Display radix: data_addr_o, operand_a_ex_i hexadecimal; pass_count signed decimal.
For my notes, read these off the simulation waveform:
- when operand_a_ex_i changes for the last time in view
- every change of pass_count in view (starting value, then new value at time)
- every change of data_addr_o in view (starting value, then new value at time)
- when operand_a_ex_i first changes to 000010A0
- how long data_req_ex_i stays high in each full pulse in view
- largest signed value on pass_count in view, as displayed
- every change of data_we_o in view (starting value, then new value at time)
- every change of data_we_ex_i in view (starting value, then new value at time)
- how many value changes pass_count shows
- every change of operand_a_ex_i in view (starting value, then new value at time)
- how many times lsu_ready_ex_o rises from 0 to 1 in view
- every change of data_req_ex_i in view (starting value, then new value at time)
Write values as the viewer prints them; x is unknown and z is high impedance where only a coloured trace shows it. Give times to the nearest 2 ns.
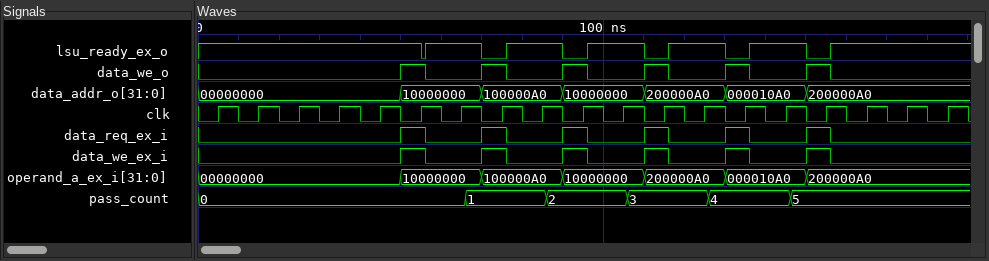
150 ns
0, 1 at 66 ns, 2 at 86 ns, 3 at 106 ns, 4 at 126 ns, 5 at 146 ns
00000000, 10000000 at 50 ns, 100000A0 at 70 ns, 10000000 at 90 ns, 200000A0 at 110 ns, 000010A0 at 130 ns, 200000A0 at 150 ns
130 ns
6 ns, 6 ns, 6 ns, 6 ns, 6 ns, 6 ns
5
0, 1 at 50 ns, 0 at 56 ns, 1 at 70 ns, 0 at 76 ns, 1 at 90 ns, 0 at 96 ns, 1 at 110 ns, 0 at 116 ns, 1 at 130 ns, 0 at 136 ns, 1 at 150 ns, 0 at 156 ns
0, 1 at 50 ns, 0 at 56 ns, 1 at 70 ns, 0 at 76 ns, 1 at 90 ns, 0 at 96 ns, 1 at 110 ns, 0 at 116 ns, 1 at 130 ns, 0 at 136 ns, 1 at 150 ns, 0 at 156 ns
5
00000000, 10000000 at 50 ns, 100000A0 at 70 ns, 10000000 at 90 ns, 200000A0 at 110 ns, 000010A0 at 130 ns, 200000A0 at 150 ns
6
0, 1 at 50 ns, 0 at 56 ns, 1 at 70 ns, 0 at 76 ns, 1 at 90 ns, 0 at 96 ns, 1 at 110 ns, 0 at 116 ns, 1 at 130 ns, 0 at 136 ns, 1 at 150 ns, 0 at 156 ns
